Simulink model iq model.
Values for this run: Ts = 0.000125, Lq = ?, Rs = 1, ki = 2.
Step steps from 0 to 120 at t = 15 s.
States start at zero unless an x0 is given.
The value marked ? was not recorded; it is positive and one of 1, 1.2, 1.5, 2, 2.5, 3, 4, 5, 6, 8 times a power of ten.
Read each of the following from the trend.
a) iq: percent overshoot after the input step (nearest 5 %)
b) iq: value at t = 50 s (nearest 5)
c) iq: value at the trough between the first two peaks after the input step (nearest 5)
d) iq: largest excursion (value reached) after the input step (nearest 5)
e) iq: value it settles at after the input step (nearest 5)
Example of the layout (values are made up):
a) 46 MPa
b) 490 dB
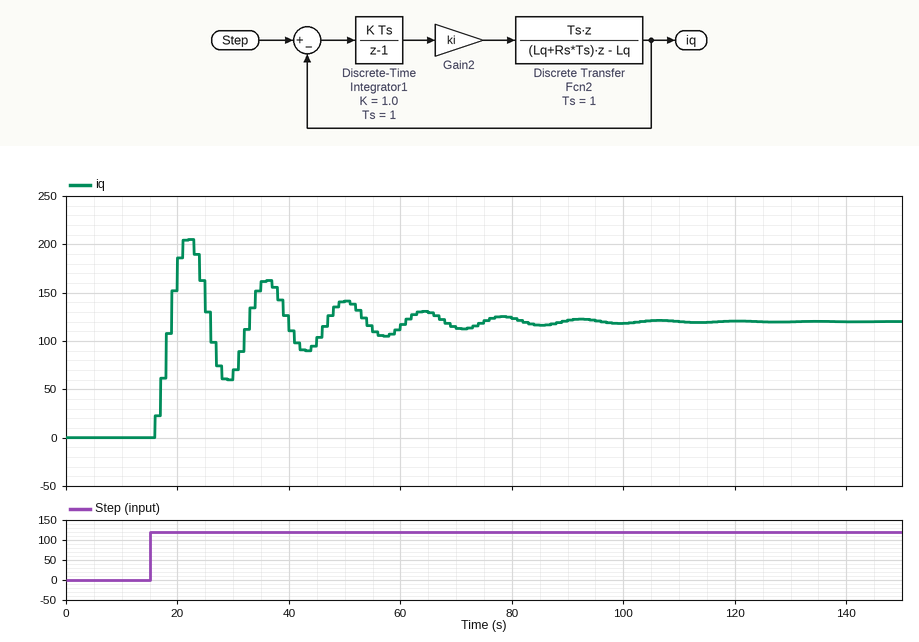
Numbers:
a) 70 %
b) 140
c) 60
d) 205
e) 120
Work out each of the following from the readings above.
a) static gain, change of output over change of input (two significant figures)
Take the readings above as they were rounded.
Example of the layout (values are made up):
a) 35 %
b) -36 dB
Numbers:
a) 1.0
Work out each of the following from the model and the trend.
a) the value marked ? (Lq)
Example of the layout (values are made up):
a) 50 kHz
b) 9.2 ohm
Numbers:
a) 0.0012
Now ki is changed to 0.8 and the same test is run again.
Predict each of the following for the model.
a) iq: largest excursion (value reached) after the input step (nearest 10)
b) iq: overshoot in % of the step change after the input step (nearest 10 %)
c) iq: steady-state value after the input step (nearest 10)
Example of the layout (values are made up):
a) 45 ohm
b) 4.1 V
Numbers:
a) 190
b) 60 %
c) 120
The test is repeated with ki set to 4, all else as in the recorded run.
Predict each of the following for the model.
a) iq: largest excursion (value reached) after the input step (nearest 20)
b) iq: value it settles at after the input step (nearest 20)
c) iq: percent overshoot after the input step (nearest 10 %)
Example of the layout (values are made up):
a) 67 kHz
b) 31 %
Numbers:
a) 220
b) 120
c) 80 %
